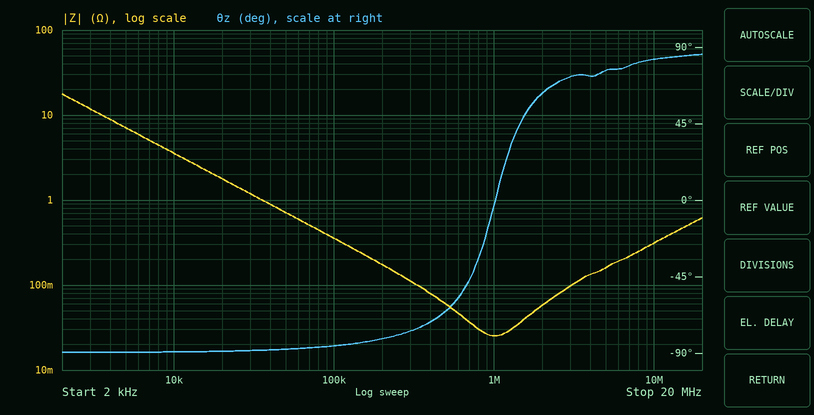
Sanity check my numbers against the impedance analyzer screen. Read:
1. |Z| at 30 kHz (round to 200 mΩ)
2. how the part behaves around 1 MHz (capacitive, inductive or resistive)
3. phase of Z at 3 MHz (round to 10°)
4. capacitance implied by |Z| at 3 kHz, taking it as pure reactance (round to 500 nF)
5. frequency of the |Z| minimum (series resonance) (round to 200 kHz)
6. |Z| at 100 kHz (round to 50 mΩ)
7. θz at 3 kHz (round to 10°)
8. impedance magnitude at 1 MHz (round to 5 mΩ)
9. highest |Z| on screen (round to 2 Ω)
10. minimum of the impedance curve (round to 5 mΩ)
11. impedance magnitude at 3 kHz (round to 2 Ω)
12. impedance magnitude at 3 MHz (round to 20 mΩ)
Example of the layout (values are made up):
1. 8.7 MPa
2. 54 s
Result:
1. 1.2 Ω
2. resistive
3. 70°
4. 4.5 µF
5. 1.0 MHz
6. 350 mΩ
7. -90°
8. 25 mΩ
9. 18 Ω
10. 25 mΩ
11. 12 Ω
12. 100 mΩ
